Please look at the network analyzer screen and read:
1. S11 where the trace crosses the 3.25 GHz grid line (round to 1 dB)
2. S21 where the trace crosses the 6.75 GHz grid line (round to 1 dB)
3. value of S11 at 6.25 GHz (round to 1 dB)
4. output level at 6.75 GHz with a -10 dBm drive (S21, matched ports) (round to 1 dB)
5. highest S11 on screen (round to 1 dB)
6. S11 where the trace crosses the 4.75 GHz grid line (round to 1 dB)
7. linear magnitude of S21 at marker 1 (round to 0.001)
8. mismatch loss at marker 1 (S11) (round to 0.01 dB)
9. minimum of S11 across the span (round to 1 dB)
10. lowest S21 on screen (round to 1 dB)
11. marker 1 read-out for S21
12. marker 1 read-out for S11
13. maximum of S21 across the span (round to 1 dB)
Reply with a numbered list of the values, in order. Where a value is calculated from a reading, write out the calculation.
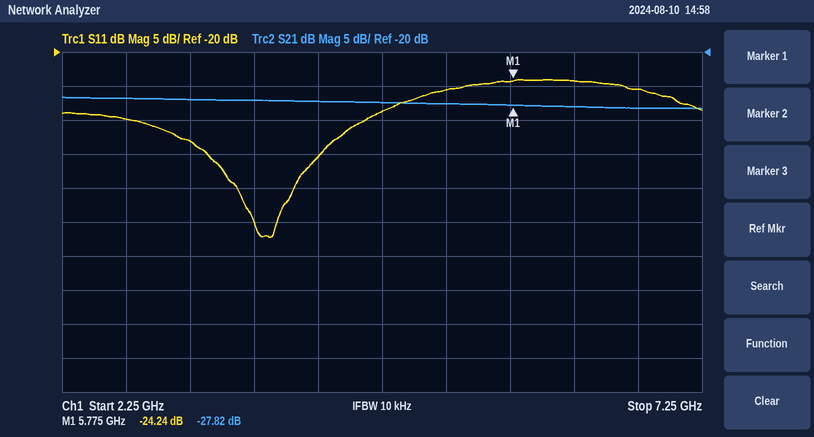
1. -33 dB
2. -28 dB
3. -24 dB
4. -10 dBm + (-28 dB) = -38 dBm
5. -24 dB
6. -29 dB
7. 10^(-27.82/20) ≈ 0.041
8. −10 log10(1 − 10^(-24.24/10)) ≈ 0.02 dB
9. -47 dB
10. -28 dB
11. -27.82 dB
12. -24.24 dB
13. -27 dB
